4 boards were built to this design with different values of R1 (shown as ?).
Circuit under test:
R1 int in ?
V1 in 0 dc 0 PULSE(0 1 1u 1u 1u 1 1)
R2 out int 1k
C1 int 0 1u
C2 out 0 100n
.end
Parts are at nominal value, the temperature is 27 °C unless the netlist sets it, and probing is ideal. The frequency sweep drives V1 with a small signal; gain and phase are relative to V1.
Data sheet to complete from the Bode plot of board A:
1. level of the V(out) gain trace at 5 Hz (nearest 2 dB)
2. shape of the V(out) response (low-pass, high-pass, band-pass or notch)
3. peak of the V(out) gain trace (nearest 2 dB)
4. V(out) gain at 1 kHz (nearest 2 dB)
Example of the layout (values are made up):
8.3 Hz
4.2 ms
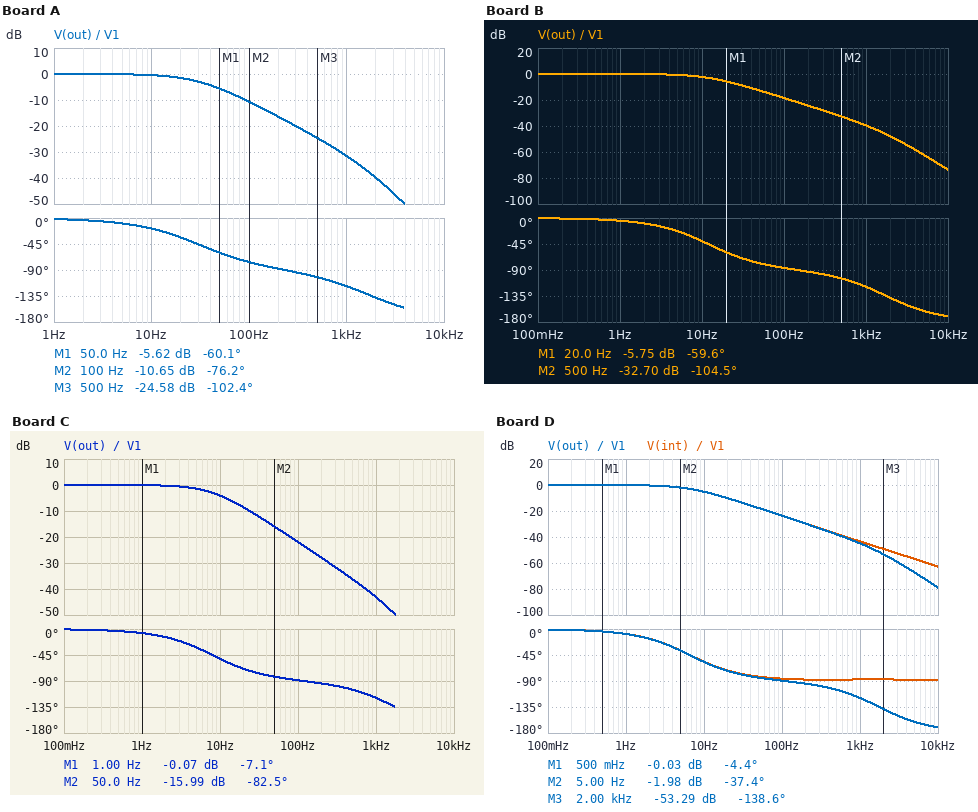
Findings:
0 dB
low-pass
0 dB
-32 dB
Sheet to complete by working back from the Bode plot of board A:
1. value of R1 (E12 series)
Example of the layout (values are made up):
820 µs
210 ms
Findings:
4.7 kΩ
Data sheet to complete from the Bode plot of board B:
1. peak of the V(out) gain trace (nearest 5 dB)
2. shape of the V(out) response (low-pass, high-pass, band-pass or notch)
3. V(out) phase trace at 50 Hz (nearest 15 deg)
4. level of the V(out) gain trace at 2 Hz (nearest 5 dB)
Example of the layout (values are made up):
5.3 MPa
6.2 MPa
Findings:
0 dB
low-pass
-75 deg
0 dB
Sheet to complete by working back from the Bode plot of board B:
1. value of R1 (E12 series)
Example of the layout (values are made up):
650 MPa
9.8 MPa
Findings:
12 kΩ
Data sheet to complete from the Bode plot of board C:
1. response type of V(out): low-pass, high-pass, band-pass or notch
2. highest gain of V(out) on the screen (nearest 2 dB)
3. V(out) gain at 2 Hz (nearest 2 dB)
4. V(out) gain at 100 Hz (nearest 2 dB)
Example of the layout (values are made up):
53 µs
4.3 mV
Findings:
low-pass
0 dB
0 dB
-22 dB
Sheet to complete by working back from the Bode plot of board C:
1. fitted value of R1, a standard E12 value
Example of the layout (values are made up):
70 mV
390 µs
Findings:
18 kΩ
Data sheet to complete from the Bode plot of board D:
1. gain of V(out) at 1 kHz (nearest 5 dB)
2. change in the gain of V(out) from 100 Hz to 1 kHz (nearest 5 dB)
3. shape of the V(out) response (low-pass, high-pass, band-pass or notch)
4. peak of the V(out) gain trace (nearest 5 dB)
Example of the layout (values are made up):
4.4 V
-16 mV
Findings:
-45 dB
-20 dB
low-pass
0 dB
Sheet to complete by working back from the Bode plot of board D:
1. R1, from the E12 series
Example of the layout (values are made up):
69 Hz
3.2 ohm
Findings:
22 kΩ
